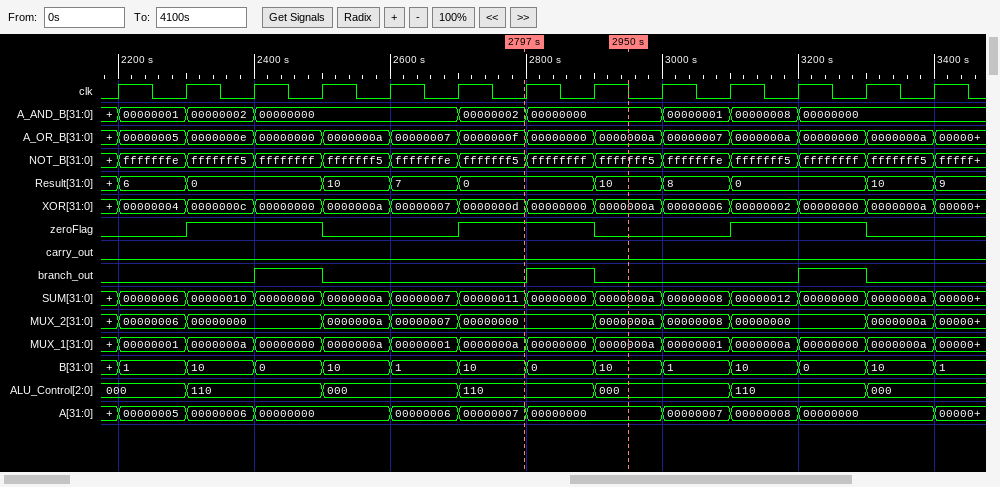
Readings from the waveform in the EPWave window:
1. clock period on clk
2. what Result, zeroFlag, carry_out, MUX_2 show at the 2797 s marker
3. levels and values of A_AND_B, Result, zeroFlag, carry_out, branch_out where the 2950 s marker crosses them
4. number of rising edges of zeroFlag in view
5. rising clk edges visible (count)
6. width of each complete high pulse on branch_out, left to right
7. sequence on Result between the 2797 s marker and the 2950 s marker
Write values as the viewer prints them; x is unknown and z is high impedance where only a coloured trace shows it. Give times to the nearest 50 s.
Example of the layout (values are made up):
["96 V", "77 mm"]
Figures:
["100 s", "Result=0, zeroFlag=1, carry_out=0, MUX_2=00000000", "A_AND_B=00000000, Result=10, zeroFlag=0, carry_out=0, branch_out=0", "3", "13", "100 s, 100 s, 100 s", "0, 10"]
